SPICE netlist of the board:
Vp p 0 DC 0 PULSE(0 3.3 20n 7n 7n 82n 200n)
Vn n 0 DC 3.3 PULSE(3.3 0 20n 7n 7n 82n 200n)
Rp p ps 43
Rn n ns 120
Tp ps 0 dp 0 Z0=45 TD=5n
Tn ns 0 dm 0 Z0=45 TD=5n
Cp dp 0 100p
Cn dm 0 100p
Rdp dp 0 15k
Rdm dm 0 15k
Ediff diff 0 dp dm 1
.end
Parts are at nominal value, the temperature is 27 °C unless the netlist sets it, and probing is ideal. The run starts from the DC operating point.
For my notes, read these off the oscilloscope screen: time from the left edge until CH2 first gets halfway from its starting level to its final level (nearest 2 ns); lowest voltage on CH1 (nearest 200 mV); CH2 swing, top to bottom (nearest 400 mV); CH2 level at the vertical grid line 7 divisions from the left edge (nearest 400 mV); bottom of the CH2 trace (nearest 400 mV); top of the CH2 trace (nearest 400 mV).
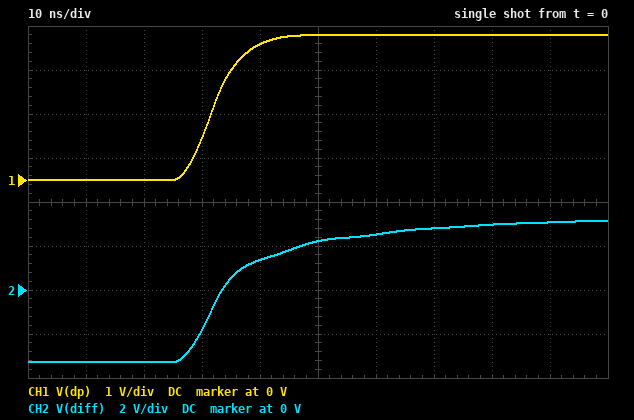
34 ns
0 V
6.4 V
2.8 V
-3.2 V
3.2 V
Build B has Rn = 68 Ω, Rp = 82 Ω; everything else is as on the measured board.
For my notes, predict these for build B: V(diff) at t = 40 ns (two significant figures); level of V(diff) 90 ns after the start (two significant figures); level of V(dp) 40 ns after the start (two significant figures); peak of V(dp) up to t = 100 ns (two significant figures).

1.1 V
3.2 V
2.1 V
3.3 V
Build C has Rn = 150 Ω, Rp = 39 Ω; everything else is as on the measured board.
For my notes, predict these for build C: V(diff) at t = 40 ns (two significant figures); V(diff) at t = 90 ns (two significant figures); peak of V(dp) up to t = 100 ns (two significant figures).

1.3 V
2.9 V
3.4 V
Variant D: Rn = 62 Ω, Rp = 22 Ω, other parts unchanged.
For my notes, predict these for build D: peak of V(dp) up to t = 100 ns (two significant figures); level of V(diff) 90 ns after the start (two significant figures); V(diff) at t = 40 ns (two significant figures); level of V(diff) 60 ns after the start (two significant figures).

4.3 V
3.3 V
3.4 V
2.9 V
